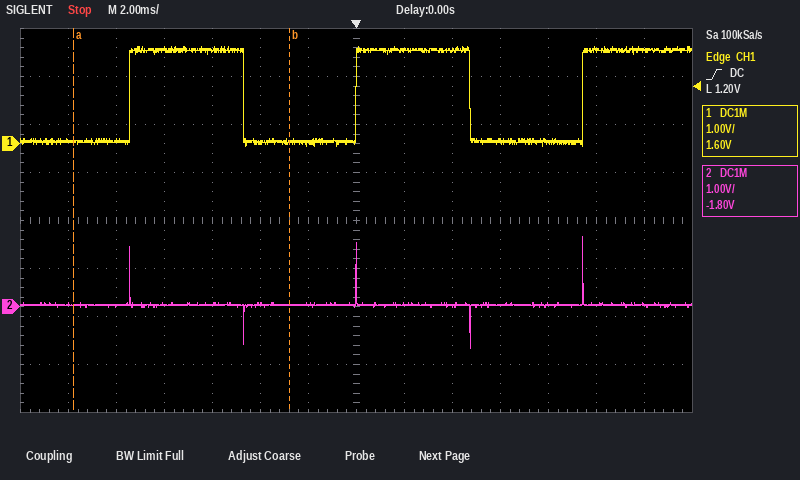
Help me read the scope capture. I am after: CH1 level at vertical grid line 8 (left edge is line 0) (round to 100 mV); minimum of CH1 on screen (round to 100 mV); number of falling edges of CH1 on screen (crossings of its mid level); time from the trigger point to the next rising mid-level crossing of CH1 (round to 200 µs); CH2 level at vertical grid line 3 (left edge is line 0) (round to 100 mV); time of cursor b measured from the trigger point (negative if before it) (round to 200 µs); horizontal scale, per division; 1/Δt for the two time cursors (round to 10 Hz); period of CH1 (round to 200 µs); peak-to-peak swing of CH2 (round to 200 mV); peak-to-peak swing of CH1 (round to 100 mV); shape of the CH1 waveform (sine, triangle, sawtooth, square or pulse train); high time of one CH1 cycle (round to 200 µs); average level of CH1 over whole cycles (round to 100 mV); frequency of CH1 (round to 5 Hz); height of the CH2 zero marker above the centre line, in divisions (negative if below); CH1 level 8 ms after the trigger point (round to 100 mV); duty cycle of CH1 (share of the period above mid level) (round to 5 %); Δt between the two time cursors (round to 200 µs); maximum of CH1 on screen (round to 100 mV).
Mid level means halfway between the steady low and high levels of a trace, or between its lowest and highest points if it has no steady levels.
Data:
1.9 V
-100 mV
2
9.4 ms
100 mV
-2.8 ms
2 ms
110 Hz
9.4 ms
2.4 V
2.1 V
square
4.8 ms
1.0 V
105 Hz
-1.8 div
0.0 V
50 %
9.0 ms
2.0 V
